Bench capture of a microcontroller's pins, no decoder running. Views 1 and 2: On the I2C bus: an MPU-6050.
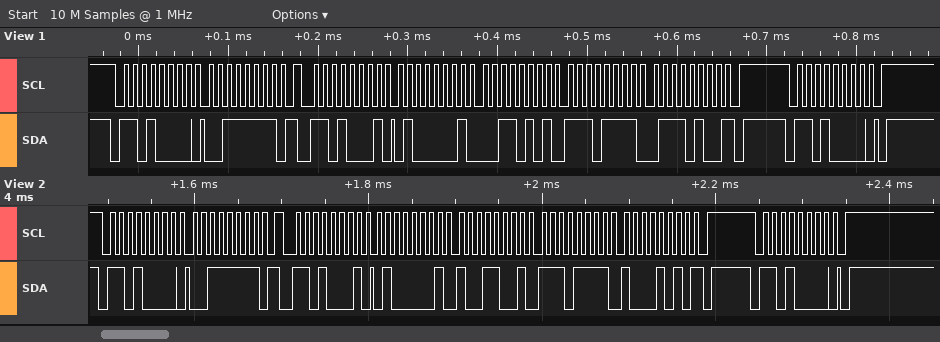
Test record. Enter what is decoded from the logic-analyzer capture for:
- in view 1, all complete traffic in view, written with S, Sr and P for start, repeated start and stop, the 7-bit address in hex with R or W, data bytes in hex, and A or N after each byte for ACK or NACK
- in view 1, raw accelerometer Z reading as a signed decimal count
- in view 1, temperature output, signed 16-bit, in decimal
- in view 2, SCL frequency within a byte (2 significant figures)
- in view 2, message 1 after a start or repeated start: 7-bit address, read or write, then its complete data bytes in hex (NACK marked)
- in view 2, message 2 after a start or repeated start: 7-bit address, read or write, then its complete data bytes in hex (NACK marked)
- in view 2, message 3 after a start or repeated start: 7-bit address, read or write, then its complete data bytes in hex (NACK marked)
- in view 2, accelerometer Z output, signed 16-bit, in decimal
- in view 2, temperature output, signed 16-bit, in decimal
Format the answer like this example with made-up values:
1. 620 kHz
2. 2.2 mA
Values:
1. S 68W A 3F A Sr 68R A 41 A 35 A EF A 74 N P S 68W A P
2. 16693
3. -4236
4. 100 kHz
5. 0x68 write: 3F
6. 0x68 read: 41 99 EF 8A NACK
7. 0x68 write
8. 16793
9. -4214
